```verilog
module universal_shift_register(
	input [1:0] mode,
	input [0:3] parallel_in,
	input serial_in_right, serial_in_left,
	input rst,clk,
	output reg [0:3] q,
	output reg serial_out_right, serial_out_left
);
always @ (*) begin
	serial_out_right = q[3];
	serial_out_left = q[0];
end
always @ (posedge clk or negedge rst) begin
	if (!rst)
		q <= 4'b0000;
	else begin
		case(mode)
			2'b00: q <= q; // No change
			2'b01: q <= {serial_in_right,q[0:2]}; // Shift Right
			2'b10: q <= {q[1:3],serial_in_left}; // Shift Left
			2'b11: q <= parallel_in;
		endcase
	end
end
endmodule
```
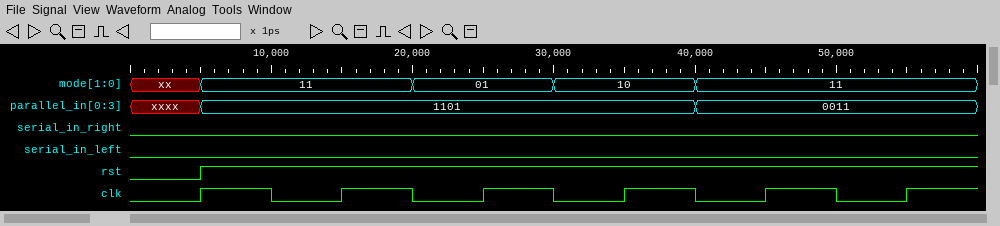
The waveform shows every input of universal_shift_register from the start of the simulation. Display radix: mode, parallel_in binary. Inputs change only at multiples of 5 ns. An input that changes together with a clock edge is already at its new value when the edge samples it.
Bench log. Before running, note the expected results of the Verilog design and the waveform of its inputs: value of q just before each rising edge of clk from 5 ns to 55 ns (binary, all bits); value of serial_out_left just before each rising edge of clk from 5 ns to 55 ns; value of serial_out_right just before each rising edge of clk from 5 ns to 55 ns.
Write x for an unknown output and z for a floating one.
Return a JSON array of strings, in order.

["0000, 1101, 1101, 0110, 1100, 0011", "0 1 1 0 1 0", "0 1 1 0 0 1"]
